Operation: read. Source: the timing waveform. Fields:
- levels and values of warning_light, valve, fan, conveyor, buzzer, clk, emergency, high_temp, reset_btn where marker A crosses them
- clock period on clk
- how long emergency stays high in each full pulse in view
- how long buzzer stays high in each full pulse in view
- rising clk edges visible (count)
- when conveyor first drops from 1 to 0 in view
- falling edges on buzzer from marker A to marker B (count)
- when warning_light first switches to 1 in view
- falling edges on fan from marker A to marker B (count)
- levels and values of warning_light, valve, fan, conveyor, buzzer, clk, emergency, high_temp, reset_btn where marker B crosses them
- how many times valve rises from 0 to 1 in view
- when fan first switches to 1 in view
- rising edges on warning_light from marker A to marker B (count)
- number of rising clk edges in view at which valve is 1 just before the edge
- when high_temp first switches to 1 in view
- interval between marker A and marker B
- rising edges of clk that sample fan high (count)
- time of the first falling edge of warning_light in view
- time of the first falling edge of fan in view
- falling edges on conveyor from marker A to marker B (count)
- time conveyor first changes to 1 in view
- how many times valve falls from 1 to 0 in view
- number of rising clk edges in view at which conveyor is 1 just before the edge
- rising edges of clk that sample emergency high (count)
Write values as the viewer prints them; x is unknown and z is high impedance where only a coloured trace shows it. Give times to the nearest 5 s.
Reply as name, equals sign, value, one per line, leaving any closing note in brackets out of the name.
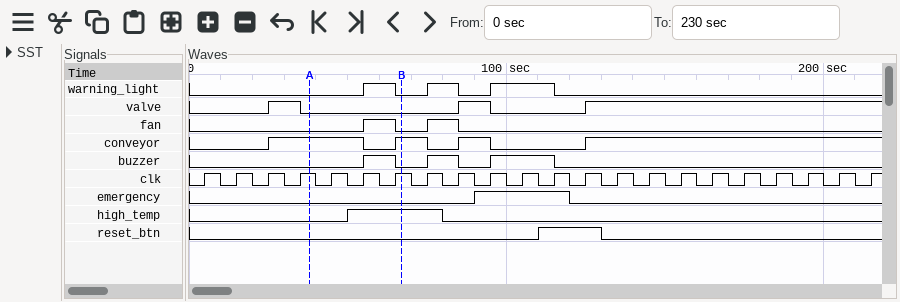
levels and values of warning_light, valve, fan, conveyor, buzzer, clk, emergency, high_temp, reset_btn where marker A crosses them = warning_light=0, valve=0, fan=0, conveyor=1, buzzer=0, clk=1, emergency=0, high_temp=0, reset_btn=0
clock period on clk = 10 s
how long emergency stays high in each full pulse in view = 30 s
how long buzzer stays high in each full pulse in view = 10 s, 10 s, 20 s
rising clk edges visible = 22
when conveyor first drops from 1 to 0 in view = 55 s
falling edges on buzzer from marker A to marker B = 1
when warning_light first switches to 1 in view = 55 s
falling edges on fan from marker A to marker B = 1
levels and values of warning_light, valve, fan, conveyor, buzzer, clk, emergency, high_temp, reset_btn where marker B crosses them = warning_light=0, valve=0, fan=0, conveyor=1, buzzer=0, clk=1, emergency=0, high_temp=1, reset_btn=0
how many times valve rises from 0 to 1 in view = 3
when fan first switches to 1 in view = 55 s
rising edges on warning_light from marker A to marker B = 1
number of rising clk edges in view at which valve is 1 just before the edge = 11
when high_temp first switches to 1 in view = 50 s
interval between marker A and marker B = 30 s
rising edges of clk that sample fan high = 2
time of the first falling edge of warning_light in view = 65 s
time of the first falling edge of fan in view = 65 s
falling edges on conveyor from marker A to marker B = 1
time conveyor first changes to 1 in view = 25 s
how many times valve falls from 1 to 0 in view = 2
number of rising clk edges in view at which conveyor is 1 just before the edge = 14
rising edges of clk that sample emergency high = 3
